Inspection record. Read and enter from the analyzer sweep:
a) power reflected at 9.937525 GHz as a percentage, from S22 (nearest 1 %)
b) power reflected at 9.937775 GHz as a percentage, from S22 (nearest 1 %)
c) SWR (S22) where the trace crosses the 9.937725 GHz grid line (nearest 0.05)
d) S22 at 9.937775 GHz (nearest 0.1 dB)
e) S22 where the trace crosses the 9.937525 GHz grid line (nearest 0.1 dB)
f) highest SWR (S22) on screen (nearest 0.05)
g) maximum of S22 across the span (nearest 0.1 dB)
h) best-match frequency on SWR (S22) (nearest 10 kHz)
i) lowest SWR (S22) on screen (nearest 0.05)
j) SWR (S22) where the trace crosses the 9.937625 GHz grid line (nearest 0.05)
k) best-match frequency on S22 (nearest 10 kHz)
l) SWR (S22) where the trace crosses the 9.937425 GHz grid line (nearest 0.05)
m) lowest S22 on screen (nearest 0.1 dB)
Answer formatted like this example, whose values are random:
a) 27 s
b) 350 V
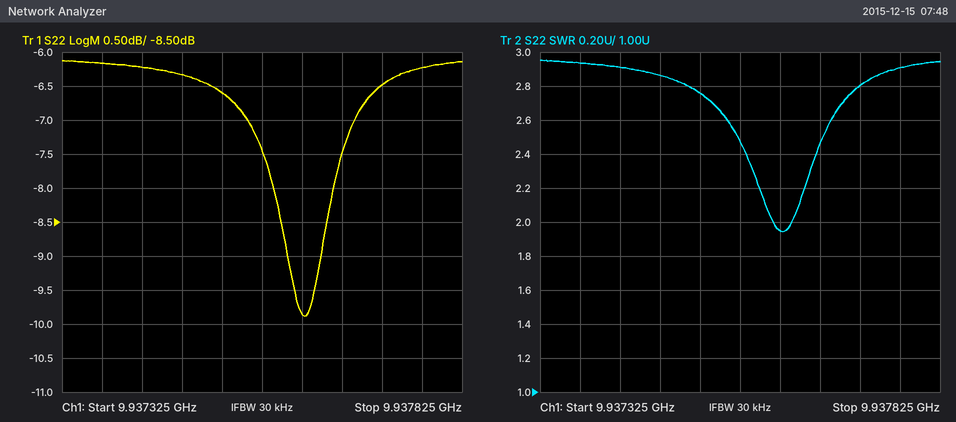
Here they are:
a) 22 %
b) 24 %
c) 2.80
d) -6.2 dB
e) -6.6 dB
f) 2.95
g) -6.1 dB
h) 9.93763 GHz
i) 1.95
j) 1.95
k) 9.93763 GHz
l) 2.90
m) -9.9 dB
